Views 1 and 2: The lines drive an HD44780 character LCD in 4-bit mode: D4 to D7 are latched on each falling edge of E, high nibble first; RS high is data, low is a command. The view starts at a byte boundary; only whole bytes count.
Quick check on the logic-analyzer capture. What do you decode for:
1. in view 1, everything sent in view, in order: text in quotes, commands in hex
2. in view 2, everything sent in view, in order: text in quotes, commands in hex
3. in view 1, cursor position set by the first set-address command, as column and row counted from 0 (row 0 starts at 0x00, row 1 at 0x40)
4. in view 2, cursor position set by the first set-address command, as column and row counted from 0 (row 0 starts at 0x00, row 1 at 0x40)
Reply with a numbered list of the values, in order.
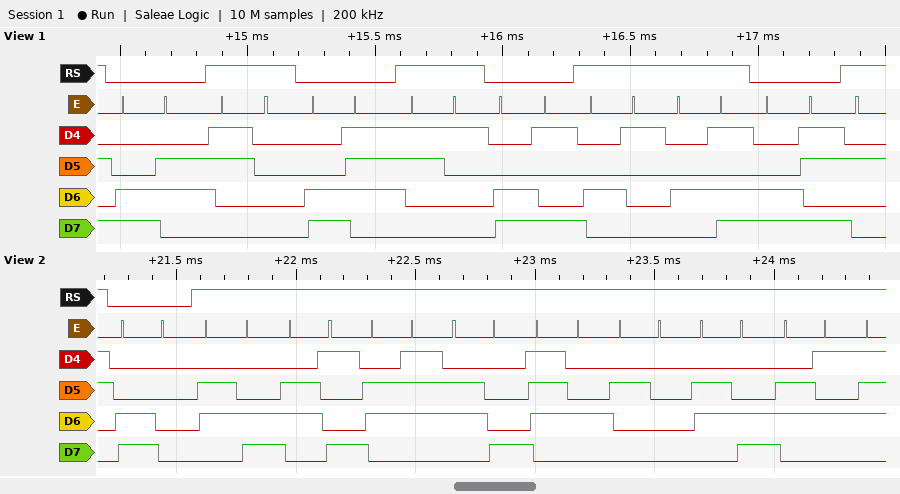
1. 0xC6 "0" 0xC7 "1" 0xC9 "AM" 0xCB
2. 0xC0 "light le"
3. column 6, row 1
4. column 0, row 1
